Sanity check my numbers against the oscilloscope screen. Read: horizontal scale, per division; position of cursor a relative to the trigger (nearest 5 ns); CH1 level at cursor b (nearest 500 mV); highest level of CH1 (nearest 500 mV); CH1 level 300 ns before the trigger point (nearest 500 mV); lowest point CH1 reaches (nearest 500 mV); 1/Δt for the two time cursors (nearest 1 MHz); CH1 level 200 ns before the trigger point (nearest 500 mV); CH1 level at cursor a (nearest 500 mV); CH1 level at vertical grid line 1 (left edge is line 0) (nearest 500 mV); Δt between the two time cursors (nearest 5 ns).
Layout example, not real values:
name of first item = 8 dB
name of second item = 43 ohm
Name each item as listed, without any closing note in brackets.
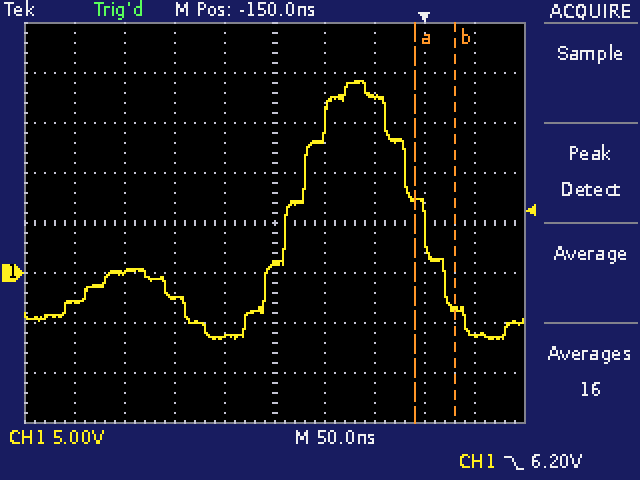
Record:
horizontal scale, per division = 50 ns
position of cursor a relative to the trigger = -10 ns
CH1 level at cursor b = -3.5 V
highest level of CH1 = 19.0 V
CH1 level 300 ns before the trigger point = 0.0 V
lowest point CH1 reaches = -6.5 V
1/Δt for the two time cursors = 25 MHz
CH1 level 200 ns before the trigger point = -6.5 V
CH1 level at cursor a = 7.5 V
CH1 level at vertical grid line 1 (left edge is line 0) = -3.0 V
Δt between the two time cursors = 40 ns
